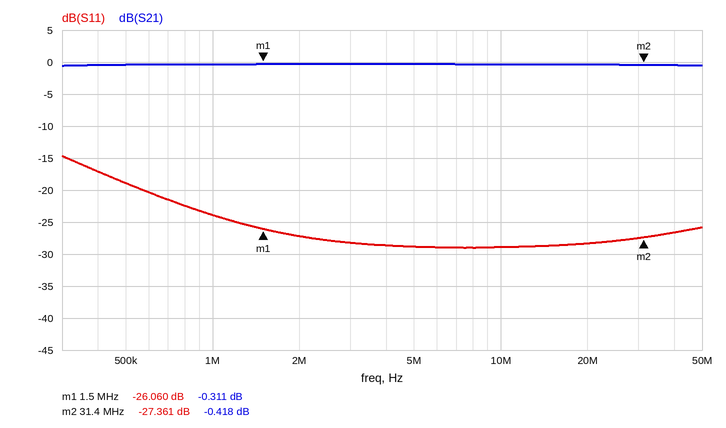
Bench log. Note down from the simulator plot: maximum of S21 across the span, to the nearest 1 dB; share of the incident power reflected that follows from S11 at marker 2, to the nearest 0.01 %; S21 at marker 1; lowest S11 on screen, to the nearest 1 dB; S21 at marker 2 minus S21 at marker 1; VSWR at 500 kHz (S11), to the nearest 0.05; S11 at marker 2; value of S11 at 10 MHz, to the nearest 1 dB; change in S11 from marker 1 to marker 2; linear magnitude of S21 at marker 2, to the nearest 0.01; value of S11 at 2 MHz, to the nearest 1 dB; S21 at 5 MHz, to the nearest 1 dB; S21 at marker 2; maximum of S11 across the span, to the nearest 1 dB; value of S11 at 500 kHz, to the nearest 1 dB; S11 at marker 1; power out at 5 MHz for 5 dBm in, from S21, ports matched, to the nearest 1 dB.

0 dB
0.18 %
-0.311 dB
-29 dB
-0.107 dB
1.25
-27.361 dB
-29 dB
-1.301 dB
0.95
-27 dB
0 dB
-0.418 dB
-15 dB
-19 dB
-26.060 dB
5 dBm
